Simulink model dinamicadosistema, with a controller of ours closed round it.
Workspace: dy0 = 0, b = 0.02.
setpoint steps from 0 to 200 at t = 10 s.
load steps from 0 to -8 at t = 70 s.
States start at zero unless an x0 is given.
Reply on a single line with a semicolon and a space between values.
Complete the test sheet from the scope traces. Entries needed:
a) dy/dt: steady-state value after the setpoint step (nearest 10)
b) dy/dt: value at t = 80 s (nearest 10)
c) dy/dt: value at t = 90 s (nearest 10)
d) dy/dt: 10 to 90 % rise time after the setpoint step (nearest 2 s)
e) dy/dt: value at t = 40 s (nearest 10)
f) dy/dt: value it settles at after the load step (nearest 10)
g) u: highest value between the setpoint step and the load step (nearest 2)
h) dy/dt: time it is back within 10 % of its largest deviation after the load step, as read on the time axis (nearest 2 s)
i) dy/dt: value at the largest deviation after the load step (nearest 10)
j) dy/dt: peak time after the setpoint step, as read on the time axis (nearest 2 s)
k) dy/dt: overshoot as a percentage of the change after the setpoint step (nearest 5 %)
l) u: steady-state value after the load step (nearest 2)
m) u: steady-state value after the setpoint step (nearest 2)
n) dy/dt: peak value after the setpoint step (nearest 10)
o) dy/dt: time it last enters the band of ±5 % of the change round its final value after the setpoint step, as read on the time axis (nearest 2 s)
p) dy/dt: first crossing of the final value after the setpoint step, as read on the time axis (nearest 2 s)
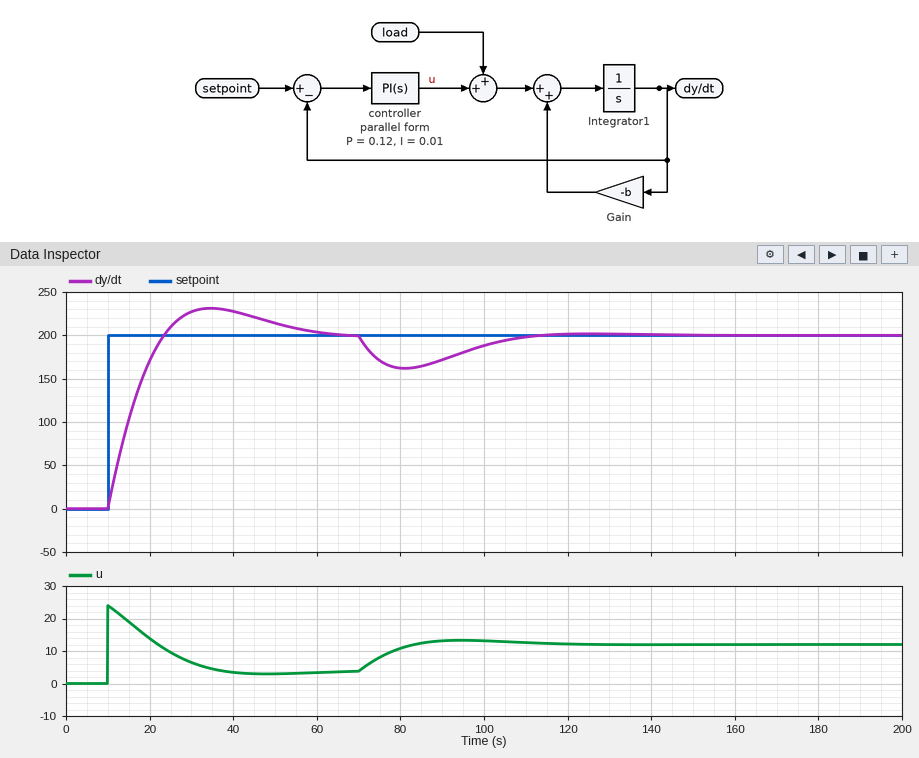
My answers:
200; 160; 170; 10 s; 230; 200; 24; 108 s; 160; 34 s; 15 %; 12; 4; 230; 54 s; 24 s
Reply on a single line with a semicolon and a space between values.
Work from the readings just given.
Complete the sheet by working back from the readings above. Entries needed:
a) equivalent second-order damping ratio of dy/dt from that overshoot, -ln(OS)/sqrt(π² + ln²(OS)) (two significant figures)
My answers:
0.52
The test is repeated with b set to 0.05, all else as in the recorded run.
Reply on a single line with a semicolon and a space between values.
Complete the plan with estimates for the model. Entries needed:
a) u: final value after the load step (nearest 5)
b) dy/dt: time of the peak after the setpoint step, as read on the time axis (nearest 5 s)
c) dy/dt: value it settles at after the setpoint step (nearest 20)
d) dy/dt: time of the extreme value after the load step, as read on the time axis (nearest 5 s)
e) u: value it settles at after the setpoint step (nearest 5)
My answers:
20; 40 s; 200; 80 s; 10
